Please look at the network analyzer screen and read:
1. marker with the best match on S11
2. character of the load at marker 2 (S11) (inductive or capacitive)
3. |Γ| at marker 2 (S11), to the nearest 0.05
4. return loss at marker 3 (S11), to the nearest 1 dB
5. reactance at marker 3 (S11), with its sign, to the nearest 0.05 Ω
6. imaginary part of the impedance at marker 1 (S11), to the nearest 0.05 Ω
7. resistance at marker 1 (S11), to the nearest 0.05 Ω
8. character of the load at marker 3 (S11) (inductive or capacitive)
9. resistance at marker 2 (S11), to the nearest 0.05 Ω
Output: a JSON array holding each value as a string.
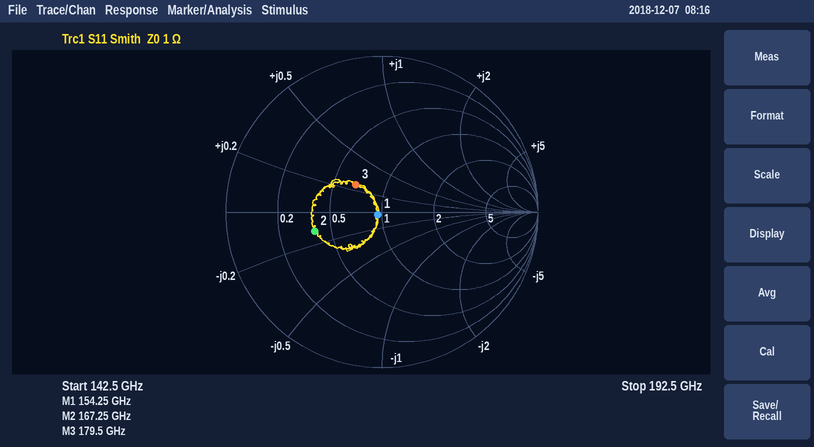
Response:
["marker 1", "capacitive", "0.45", "12 dB", "+0.25 Ω", "-0.05 Ω", "0.95 Ω", "inductive", "0.40 Ω"]
